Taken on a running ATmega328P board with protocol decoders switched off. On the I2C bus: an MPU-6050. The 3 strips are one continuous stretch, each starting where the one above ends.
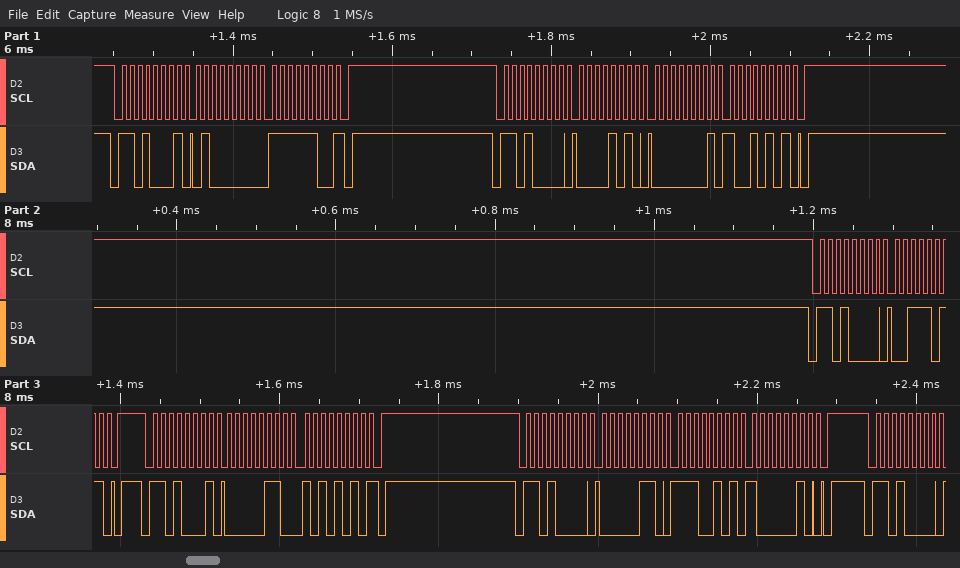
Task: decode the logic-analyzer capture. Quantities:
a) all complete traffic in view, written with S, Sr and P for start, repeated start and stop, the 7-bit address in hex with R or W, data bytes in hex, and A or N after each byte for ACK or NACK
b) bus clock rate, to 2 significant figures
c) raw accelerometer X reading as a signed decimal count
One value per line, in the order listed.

S 68R A 40 A FC N P S 68W A 0A A 01 A 95 A P S 68W A 3B A P S 68R A 06 A AA N P S 68W A 06 A E5 A 82 A P S 68W A
100 kHz
1706
